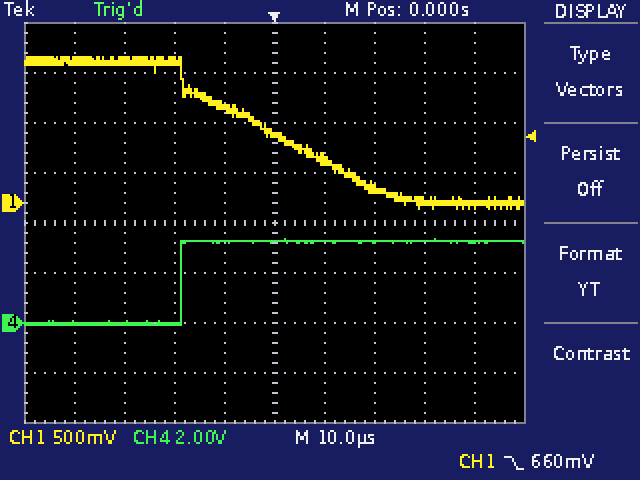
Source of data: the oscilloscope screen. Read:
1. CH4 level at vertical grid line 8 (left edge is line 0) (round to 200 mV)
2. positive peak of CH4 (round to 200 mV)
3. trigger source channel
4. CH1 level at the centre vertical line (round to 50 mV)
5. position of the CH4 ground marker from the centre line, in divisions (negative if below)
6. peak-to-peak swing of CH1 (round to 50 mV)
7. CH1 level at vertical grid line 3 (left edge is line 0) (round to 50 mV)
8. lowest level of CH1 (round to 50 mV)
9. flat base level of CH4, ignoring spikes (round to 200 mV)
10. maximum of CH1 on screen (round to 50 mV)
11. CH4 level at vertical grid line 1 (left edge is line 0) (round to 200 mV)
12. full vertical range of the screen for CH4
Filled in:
3.2 V
3.4 V
CH1
700 mV
-2.0 div
1.50 V
1.40 V
-50 mV
0.0 V
1.45 V
0.0 V
16 V
